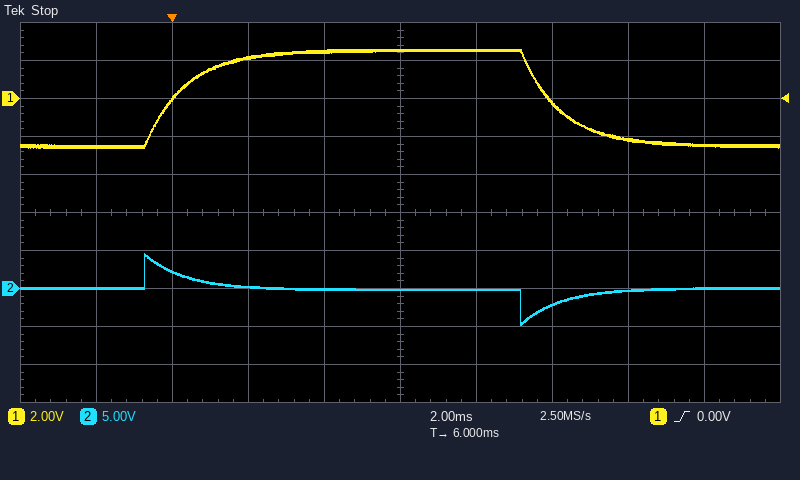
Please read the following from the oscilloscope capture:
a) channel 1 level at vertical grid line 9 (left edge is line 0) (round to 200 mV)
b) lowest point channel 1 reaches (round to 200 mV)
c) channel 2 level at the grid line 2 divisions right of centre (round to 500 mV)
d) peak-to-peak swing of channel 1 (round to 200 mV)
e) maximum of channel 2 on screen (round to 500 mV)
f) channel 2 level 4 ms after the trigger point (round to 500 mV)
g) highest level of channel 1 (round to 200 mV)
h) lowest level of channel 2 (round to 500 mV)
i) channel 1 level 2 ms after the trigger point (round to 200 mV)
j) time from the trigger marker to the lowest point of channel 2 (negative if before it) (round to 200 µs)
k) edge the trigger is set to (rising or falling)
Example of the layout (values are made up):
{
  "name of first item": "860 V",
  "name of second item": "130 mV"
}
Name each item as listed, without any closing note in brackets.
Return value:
{
  "channel 1 level at vertical grid line 9 (left edge is line 0)": "-2.4 V",
  "lowest point channel 1 reaches": "-2.6 V",
  "channel 2 level at the grid line 2 divisions right of centre": "-2.0 V",
  "peak-to-peak swing of channel 1": "5.2 V",
  "maximum of channel 2 on screen": "4.5 V",
  "channel 2 level 4 ms after the trigger point": "0.0 V",
  "highest level of channel 1": "2.6 V",
  "lowest level of channel 2": "-4.5 V",
  "channel 1 level 2 ms after the trigger point": "2.2 V",
  "time from the trigger marker to the lowest point of channel 2 (negative if before it)": "+9.2 ms",
  "edge the trigger is set to": "rising"
}
